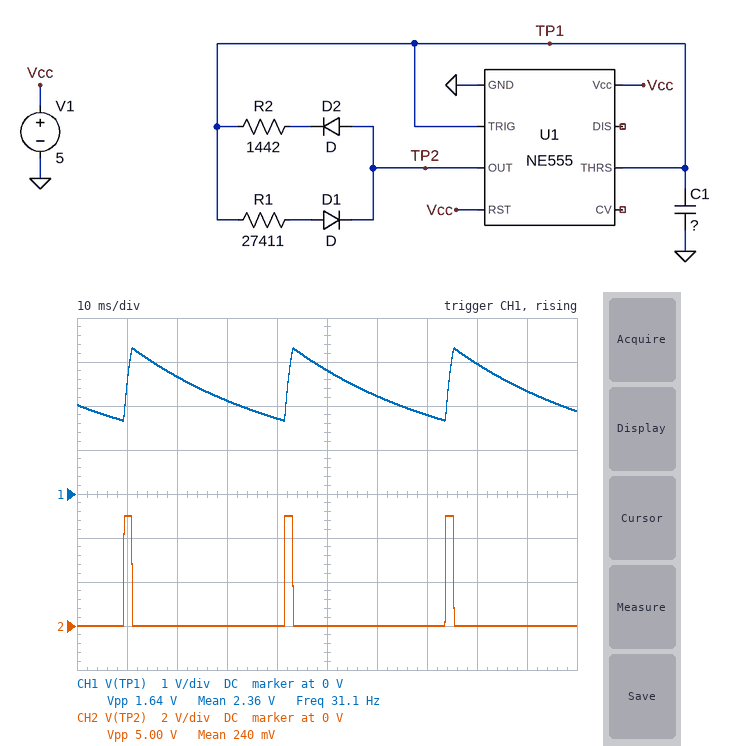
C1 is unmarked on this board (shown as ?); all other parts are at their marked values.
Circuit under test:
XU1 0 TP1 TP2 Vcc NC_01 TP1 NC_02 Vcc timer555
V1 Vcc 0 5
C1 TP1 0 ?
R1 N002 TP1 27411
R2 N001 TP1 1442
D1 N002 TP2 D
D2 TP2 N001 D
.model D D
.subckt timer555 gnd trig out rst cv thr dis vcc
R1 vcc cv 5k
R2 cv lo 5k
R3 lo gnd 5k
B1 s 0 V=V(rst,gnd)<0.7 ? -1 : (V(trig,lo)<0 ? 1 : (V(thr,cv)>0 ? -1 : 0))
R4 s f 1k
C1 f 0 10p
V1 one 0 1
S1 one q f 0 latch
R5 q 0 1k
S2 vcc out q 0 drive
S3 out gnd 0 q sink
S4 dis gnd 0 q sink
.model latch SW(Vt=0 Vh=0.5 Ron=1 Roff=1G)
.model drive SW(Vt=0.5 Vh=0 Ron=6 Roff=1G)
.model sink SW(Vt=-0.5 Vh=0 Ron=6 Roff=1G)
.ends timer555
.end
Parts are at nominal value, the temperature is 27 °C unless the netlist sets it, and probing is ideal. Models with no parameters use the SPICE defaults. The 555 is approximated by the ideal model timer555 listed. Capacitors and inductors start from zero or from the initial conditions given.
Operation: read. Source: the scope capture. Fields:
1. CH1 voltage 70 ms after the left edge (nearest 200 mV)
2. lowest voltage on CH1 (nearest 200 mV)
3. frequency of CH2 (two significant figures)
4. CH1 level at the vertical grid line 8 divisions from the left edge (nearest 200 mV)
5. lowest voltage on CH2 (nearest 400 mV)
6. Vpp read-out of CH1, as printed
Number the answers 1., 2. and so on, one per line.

1. 1.8 V
2. 1.6 V
3. 31 Hz
4. 3.0 V
5. 0 V
6. 1.64 V
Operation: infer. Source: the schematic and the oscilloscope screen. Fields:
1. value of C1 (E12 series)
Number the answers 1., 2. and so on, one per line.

1. 1.2 µF
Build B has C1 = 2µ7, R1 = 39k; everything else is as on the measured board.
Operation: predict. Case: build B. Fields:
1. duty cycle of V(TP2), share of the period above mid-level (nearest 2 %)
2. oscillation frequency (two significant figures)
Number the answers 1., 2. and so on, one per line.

1. 4 %
2. 9.9 Hz
